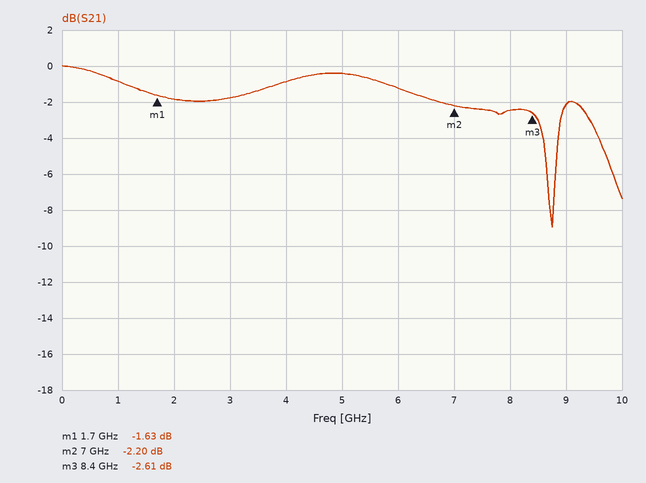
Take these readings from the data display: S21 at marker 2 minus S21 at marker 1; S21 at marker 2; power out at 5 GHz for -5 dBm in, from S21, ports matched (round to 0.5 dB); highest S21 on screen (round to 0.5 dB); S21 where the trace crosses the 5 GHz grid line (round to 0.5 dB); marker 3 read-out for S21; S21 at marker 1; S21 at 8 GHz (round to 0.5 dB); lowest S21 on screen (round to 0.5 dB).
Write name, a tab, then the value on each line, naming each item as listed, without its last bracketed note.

S21 at marker 2 minus S21 at marker 1	-0.57 dB
S21 at marker 2	-2.20 dB
power out at 5 GHz for -5 dBm in, from S21, ports matched	-5.5 dBm
highest S21 on screen	0.0 dB
S21 where the trace crosses the 5 GHz grid line	-0.5 dB
marker 3 read-out for S21	-2.61 dB
S21 at marker 1	-1.63 dB
S21 at 8 GHz	-2.5 dB
lowest S21 on screen	-9.0 dB
